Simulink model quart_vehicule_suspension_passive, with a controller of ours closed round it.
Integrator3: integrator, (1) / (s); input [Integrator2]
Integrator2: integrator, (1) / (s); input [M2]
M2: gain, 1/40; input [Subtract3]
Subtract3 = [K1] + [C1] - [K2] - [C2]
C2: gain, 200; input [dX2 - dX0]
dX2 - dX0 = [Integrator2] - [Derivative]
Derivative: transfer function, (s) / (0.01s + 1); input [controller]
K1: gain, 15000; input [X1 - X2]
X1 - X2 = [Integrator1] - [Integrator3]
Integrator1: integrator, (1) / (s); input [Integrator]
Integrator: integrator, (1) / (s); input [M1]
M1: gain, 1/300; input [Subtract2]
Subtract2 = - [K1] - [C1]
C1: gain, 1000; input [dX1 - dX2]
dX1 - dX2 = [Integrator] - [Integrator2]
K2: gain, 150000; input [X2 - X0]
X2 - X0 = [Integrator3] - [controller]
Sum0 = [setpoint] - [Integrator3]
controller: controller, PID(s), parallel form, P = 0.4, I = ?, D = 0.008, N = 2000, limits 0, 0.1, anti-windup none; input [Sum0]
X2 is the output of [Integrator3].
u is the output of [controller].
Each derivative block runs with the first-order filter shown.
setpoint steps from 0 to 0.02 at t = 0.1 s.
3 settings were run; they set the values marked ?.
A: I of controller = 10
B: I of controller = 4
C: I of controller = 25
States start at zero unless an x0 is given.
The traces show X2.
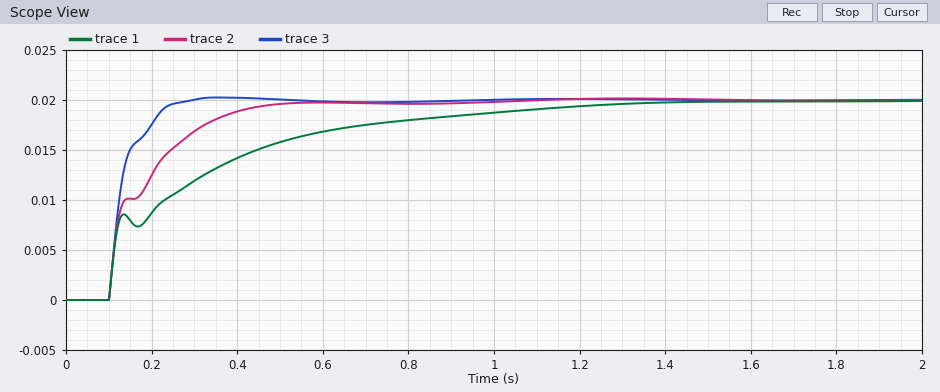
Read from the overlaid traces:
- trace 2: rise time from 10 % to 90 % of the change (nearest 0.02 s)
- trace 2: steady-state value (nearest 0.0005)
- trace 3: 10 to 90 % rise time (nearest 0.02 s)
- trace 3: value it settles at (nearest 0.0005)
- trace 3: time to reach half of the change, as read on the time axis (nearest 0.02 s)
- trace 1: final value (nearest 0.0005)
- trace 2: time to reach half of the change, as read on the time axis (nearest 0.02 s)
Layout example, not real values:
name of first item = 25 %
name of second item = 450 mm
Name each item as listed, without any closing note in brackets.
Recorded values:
trace 2: rise time from 10 % to 90 % of the change = 0.24 s
trace 2: steady-state value = 0.0200
trace 3: 10 to 90 % rise time = 0.10 s
trace 3: value it settles at = 0.0200
trace 3: time to reach half of the change, as read on the time axis = 0.12 s
trace 1: final value = 0.0200
trace 2: time to reach half of the change, as read on the time axis = 0.14 s
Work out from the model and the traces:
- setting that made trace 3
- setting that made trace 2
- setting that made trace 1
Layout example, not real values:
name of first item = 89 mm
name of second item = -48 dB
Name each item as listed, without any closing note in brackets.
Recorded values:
setting that made trace 3 = C
setting that made trace 2 = A
setting that made trace 1 = B
